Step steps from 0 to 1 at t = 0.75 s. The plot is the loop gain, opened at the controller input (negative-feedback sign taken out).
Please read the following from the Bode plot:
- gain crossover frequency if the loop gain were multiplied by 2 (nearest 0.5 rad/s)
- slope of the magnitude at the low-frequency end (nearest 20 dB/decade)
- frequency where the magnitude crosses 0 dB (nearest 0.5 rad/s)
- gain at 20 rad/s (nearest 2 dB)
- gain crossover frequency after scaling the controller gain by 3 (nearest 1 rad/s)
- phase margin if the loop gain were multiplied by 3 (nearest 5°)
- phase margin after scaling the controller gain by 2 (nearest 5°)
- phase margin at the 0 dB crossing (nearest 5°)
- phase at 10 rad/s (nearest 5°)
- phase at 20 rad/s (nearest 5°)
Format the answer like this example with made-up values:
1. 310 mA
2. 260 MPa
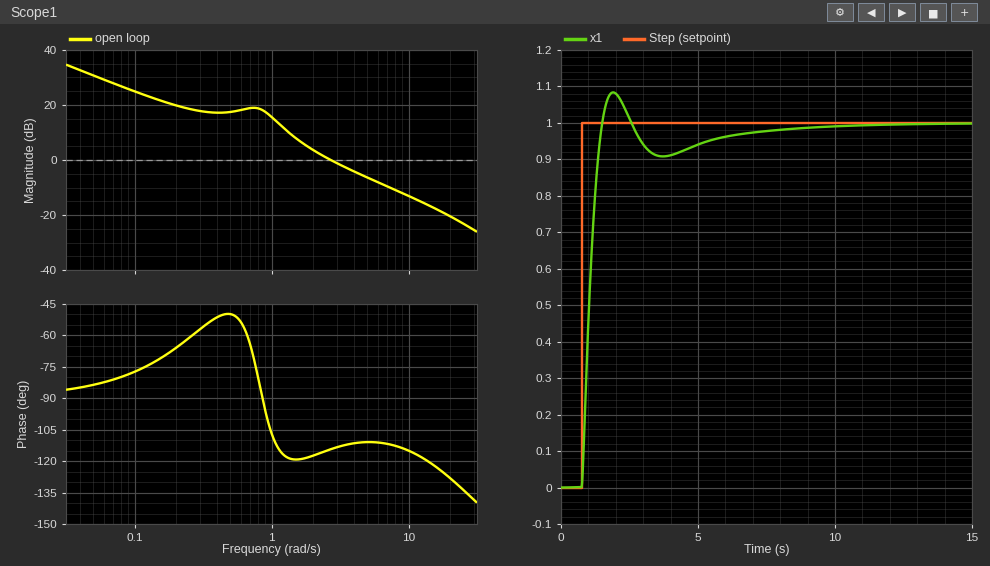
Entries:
1. 5.0 rad/s
2. -20 dB/decade
3. 2.5 rad/s
4. -20 dB
5. 7 rad/s
6. 70°
7. 70°
8. 65°
9. -115°
10. -130°
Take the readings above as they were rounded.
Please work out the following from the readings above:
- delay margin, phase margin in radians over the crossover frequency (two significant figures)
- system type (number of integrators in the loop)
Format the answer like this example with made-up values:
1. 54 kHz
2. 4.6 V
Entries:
1. 0.45 s
2. 1
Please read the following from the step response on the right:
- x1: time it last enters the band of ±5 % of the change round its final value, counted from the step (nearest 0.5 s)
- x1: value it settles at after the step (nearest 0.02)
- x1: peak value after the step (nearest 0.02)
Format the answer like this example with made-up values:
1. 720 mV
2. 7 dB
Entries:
1. 4.5 s
2. 1.00
3. 1.08
